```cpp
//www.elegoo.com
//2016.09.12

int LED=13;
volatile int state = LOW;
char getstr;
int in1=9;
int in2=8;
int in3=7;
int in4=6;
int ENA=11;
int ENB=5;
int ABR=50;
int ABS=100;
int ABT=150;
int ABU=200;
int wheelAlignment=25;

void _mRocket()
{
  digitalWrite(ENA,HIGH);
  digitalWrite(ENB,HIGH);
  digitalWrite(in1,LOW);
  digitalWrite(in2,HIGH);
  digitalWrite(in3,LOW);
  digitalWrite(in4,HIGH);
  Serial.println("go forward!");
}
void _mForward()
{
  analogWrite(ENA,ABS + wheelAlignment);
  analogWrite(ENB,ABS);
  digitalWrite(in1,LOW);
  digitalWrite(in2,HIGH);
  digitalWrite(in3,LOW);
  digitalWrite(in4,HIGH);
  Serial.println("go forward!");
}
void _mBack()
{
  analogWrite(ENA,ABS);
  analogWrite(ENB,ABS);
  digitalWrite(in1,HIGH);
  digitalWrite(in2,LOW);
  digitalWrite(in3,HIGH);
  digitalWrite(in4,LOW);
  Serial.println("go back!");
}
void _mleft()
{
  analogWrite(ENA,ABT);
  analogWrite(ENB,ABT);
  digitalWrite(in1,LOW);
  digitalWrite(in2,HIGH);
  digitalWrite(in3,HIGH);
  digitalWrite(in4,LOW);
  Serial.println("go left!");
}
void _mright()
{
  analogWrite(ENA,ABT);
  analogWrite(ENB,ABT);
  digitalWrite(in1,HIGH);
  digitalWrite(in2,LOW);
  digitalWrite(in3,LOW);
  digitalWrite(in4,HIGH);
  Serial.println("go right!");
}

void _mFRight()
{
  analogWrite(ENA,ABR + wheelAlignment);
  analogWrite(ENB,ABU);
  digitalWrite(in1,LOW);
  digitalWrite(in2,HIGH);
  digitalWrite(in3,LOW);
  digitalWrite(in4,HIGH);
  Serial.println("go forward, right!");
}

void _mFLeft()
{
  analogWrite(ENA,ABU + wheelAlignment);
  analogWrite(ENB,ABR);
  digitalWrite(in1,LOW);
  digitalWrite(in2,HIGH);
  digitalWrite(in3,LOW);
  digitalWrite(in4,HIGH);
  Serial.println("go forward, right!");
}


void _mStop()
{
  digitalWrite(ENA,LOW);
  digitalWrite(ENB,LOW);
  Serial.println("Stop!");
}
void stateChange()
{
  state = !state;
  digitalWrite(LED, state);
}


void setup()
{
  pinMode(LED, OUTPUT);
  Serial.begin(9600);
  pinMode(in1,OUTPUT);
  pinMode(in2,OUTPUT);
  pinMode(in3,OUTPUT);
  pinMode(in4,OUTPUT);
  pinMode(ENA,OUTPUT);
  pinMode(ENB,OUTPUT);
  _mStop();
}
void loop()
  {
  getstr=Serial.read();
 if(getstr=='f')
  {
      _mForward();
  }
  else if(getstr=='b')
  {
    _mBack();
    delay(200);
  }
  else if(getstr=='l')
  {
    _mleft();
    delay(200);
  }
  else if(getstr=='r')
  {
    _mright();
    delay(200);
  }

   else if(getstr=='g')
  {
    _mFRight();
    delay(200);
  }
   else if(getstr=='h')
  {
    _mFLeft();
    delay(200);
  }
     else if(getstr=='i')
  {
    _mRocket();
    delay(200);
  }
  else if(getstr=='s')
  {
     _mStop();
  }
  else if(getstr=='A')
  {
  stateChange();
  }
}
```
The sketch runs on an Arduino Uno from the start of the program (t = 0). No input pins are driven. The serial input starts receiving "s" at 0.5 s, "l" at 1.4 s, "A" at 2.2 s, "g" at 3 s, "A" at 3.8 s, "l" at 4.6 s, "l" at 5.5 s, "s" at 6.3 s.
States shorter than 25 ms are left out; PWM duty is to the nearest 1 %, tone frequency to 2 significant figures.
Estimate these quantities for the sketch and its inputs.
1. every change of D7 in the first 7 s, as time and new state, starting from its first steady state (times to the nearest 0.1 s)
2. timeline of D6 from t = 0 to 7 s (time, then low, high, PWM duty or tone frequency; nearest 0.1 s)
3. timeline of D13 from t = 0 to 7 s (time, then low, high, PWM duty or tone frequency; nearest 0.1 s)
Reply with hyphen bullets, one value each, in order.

- 0 s low; 1.4 s high; 3 s low; 4.6 s high
- 0 s low; 3 s high; 4.6 s low
- 0 s low; 2.2 s high; 3.8 s low
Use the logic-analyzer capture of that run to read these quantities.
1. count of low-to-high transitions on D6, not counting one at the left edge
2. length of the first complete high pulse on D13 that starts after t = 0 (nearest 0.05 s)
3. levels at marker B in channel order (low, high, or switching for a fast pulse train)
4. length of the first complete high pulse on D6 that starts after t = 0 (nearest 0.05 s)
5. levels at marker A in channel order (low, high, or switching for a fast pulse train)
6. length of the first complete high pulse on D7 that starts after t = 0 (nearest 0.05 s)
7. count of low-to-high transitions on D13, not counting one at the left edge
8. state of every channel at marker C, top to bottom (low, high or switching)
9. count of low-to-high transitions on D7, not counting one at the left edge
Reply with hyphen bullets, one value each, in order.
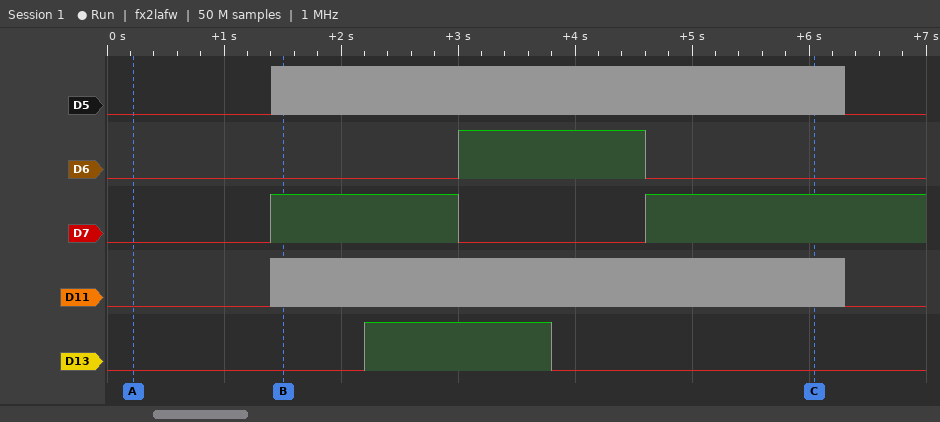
- 1
- 1.60 s
- D5 switching, D6 low, D7 high, D11 switching, D13 low
- 1.60 s
- D5 low, D6 low, D7 low, D11 low, D13 low
- 1.60 s
- 1
- D5 switching, D6 low, D7 high, D11 switching, D13 low
- 2
